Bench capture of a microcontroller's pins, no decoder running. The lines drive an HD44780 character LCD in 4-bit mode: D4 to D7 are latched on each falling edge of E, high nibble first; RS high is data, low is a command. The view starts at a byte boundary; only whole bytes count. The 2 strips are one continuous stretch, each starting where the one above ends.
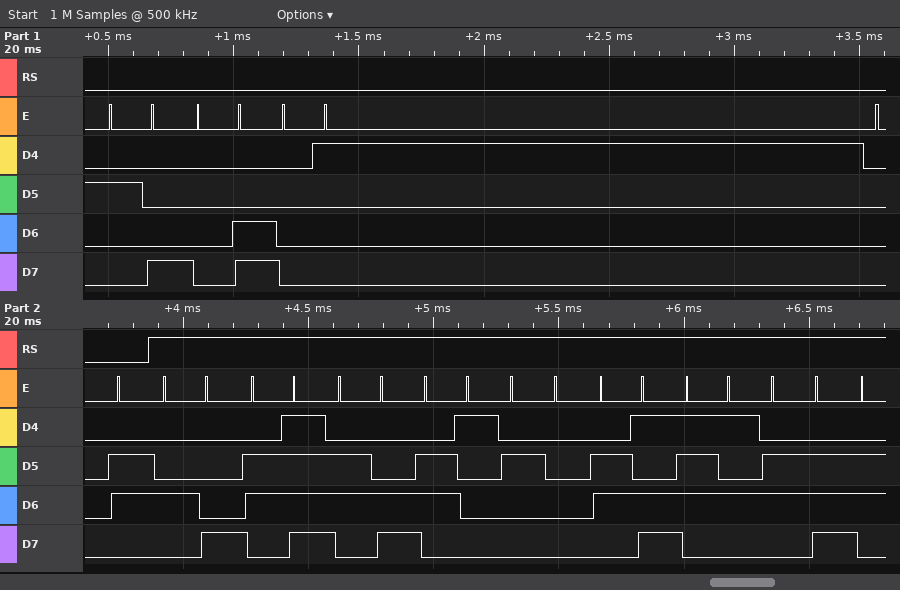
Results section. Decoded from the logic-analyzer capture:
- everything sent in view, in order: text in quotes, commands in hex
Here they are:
0x28 0x0C 0x01 0x06 "Hola mun"
